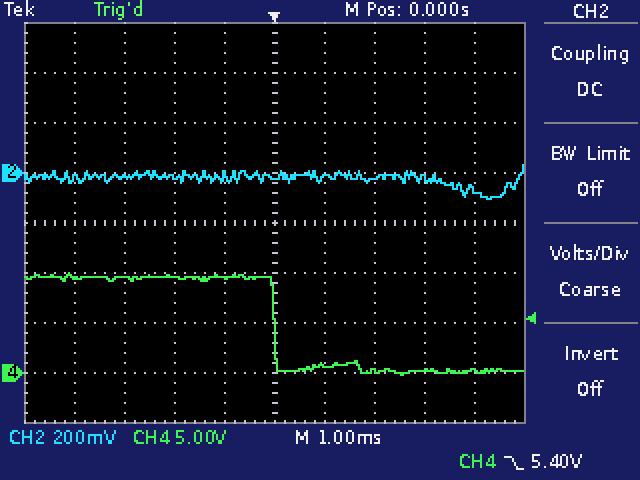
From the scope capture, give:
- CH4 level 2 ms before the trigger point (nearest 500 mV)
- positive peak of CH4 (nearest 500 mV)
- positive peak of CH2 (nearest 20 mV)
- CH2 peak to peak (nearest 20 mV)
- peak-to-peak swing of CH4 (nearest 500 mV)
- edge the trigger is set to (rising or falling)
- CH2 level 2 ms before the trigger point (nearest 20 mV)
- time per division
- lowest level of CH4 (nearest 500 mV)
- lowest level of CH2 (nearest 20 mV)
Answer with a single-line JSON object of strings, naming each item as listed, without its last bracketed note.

{"CH4 level 2 ms before the trigger point": "9.5 V", "positive peak of CH4": "10.0 V", "positive peak of CH2": "40 mV", "CH2 peak to peak": "140 mV", "peak-to-peak swing of CH4": "10.0 V", "edge the trigger is set to": "falling", "CH2 level 2 ms before the trigger point": "-20 mV", "time per division": "1 ms", "lowest level of CH4": "0.0 V", "lowest level of CH2": "-100 mV"}
